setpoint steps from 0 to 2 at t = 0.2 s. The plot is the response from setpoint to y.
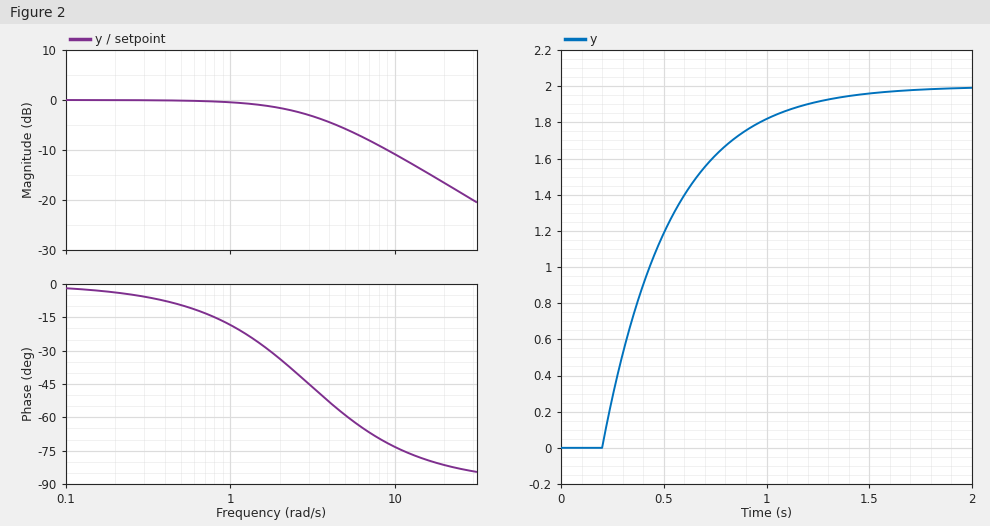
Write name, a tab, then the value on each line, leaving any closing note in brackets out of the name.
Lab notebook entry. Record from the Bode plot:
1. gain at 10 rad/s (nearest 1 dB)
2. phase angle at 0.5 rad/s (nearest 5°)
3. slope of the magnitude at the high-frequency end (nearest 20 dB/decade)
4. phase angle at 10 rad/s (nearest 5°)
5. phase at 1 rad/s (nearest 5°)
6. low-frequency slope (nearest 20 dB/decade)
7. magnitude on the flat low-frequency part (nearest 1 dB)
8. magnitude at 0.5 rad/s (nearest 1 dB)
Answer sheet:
gain at 10 rad/s	-11 dB
phase angle at 0.5 rad/s	-10°
slope of the magnitude at the high-frequency end	-20 dB/decade
phase angle at 10 rad/s	-75°
phase at 1 rad/s	-20°
low-frequency slope	0 dB/decade
magnitude on the flat low-frequency part	0 dB
magnitude at 0.5 rad/s	0 dB
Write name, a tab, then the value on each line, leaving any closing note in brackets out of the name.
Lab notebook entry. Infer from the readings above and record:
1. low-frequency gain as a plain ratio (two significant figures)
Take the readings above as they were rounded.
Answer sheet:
low-frequency gain as a plain ratio	1.0
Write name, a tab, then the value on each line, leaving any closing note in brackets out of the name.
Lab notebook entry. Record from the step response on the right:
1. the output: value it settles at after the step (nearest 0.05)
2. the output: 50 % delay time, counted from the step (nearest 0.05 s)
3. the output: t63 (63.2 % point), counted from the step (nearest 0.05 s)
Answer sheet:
the output: value it settles at after the step	2.00
the output: 50 % delay time, counted from the step	0.25 s
the output: t63 (63.2 % point), counted from the step	0.35 s
